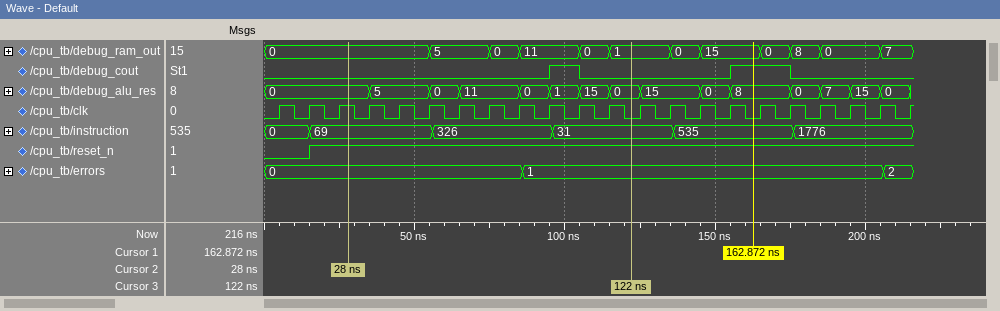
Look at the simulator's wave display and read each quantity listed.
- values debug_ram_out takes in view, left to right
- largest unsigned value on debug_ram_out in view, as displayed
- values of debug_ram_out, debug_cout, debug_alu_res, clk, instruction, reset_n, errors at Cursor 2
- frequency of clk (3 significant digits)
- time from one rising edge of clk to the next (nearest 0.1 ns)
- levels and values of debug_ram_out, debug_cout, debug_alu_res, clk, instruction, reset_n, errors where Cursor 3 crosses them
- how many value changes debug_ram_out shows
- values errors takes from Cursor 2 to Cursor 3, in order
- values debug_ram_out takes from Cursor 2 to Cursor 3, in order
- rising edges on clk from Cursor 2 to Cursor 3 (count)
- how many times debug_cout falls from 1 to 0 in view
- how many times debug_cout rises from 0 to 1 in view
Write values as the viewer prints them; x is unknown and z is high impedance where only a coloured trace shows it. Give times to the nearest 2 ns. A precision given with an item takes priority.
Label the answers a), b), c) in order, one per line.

a) 0, 5, 0, 11, 0, 1, 0, 15, 0, 8, 0, 7
b) 15
c) debug_ram_out=0, debug_cout=0, debug_alu_res=0, clk=1, instruction=69, reset_n=1, errors=0
d) 100 MHz
e) 10 ns
f) debug_ram_out=1, debug_cout=0, debug_alu_res=0, clk=0, instruction=31, reset_n=1, errors=1
g) 11
h) 0, 1
i) 0, 5, 0, 11, 0, 1
j) 9
k) 2
l) 2
